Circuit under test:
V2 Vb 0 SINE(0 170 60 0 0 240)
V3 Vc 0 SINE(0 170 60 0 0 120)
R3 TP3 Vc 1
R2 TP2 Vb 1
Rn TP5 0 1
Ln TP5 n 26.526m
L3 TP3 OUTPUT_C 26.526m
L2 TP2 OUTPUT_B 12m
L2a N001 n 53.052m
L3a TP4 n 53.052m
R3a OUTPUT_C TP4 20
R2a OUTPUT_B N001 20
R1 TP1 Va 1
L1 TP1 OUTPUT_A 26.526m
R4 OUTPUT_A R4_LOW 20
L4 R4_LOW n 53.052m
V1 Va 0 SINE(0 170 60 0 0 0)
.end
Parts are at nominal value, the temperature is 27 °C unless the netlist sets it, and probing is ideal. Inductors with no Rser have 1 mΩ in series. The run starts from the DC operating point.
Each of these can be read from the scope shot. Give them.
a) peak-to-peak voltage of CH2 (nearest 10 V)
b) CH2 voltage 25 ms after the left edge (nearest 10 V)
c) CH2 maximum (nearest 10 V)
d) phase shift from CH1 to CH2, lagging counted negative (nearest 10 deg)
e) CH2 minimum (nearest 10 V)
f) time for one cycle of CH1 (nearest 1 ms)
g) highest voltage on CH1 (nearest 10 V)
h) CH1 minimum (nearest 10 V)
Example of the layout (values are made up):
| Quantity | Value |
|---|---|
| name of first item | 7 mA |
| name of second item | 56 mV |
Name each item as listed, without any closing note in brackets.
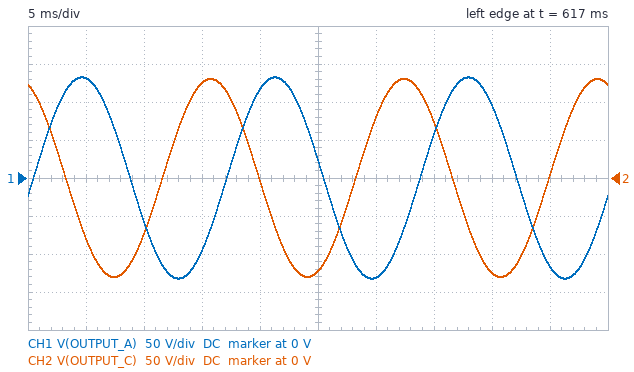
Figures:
| Quantity | Value |
|---|---|
| peak-to-peak voltage of CH2 | 260 V |
| CH2 voltage 25 ms after the left edge | -120 V |
| CH2 maximum | 130 V |
| phase shift from CH1 to CH2, lagging counted negative | 120 deg |
| CH2 minimum | -130 V |
| time for one cycle of CH1 | 17 ms |
| highest voltage on CH1 | 130 V |
| CH1 minimum | -130 V |
